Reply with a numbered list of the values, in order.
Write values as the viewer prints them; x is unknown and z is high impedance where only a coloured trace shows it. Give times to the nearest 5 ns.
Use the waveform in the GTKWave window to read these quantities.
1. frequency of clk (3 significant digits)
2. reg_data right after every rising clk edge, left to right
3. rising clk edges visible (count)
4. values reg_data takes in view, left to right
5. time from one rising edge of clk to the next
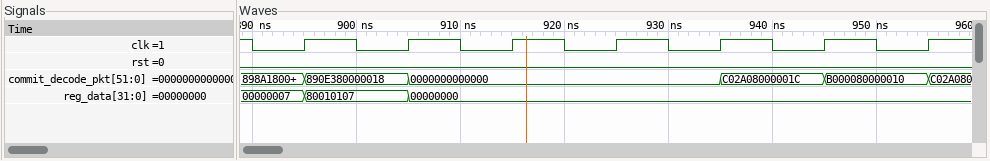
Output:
1. 100 MHz
2. 80010107, 00000000, 00000000, 00000000, 00000000, 00000000, 00000000
3. 7
4. 00000007, 80010107, 00000000
5. 10 ns
